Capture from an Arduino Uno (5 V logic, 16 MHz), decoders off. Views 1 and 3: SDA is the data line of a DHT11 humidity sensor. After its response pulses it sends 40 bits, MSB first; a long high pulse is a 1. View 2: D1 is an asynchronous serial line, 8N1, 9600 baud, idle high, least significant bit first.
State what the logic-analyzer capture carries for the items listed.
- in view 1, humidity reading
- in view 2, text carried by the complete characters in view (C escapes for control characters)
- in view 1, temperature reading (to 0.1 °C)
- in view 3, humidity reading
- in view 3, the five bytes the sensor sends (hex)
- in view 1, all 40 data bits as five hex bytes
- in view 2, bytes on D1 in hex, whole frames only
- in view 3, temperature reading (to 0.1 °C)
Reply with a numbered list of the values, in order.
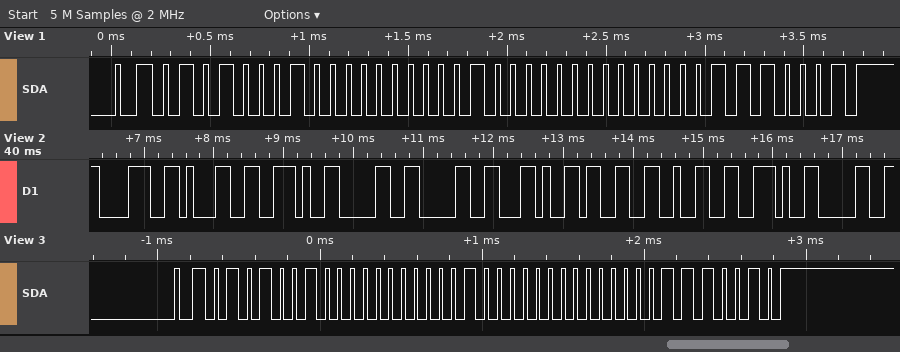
1. 81 %
2. "81.00,32.0"
3. 32.0 °C
4. 82 %
5. 52 00 20 00 72
6. 51 00 20 00 71
7. 38 31 2E 30 30 2C 33 32 2E 30
8. 32.0 °C
